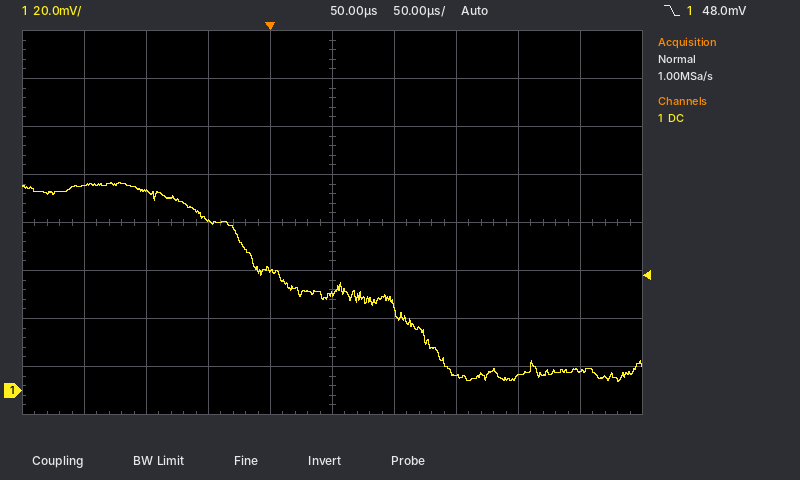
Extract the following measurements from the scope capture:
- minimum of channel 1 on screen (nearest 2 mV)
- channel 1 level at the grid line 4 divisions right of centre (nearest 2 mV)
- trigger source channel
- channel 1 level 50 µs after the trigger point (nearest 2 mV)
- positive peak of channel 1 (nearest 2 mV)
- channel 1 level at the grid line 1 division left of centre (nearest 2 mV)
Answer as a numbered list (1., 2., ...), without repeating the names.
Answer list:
1. 4 mV
2. 8 mV
3. channel 1
4. 40 mV
5. 86 mV
6. 50 mV
